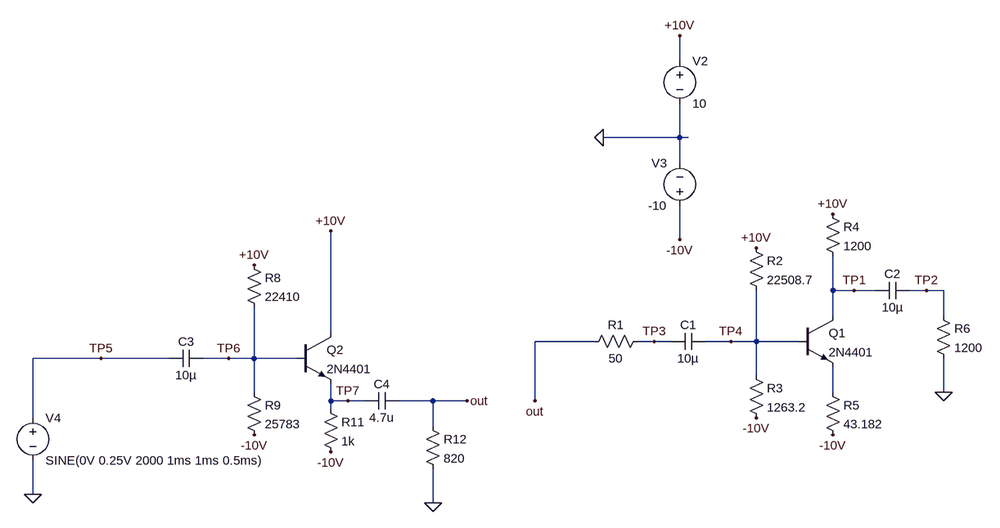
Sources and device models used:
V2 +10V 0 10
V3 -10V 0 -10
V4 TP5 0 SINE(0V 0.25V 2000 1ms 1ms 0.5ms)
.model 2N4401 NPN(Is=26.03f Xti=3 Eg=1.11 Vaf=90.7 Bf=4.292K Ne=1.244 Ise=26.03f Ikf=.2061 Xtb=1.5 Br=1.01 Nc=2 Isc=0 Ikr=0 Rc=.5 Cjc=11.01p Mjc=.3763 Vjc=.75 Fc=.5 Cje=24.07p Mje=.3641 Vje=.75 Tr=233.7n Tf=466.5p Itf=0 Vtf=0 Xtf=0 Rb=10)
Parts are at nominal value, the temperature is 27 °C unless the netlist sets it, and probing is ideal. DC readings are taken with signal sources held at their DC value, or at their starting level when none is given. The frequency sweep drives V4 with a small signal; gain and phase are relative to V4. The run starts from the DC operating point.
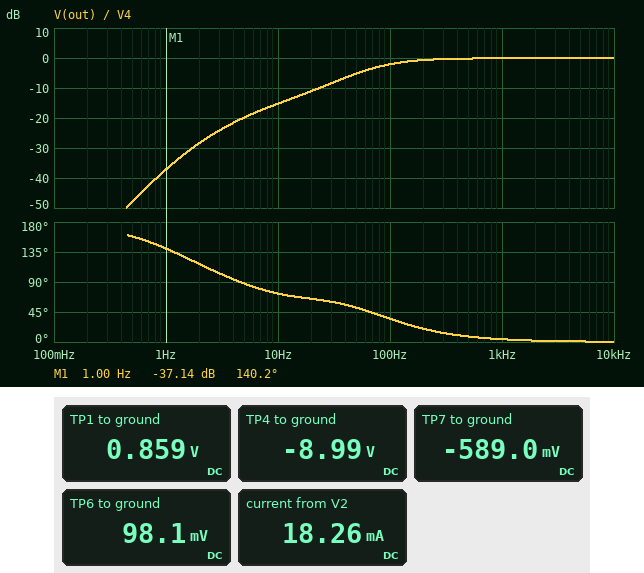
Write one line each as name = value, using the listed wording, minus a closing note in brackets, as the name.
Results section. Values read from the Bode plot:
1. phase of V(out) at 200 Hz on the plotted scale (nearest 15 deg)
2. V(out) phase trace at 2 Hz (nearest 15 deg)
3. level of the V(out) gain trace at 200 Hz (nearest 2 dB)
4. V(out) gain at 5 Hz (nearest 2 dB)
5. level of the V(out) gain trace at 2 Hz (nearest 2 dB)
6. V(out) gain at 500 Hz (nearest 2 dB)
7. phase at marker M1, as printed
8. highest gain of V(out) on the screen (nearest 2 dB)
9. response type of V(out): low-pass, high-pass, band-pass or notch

phase of V(out) at 200 Hz on the plotted scale = 15 deg
V(out) phase trace at 2 Hz = 120 deg
level of the V(out) gain trace at 200 Hz = 0 dB
V(out) gain at 5 Hz = -20 dB
level of the V(out) gain trace at 2 Hz = -28 dB
V(out) gain at 500 Hz = 0 dB
phase at marker M1, as printed = 140.2 deg
highest gain of V(out) on the screen = 0 dB
response type of V(out): low-pass, high-pass, band-pass or notch = high-pass
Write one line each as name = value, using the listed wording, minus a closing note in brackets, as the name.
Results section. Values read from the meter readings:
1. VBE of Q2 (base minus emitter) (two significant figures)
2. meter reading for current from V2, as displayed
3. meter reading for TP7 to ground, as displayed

VBE of Q2 (base minus emitter) = 690 mV
meter reading for current from V2, as displayed = 18.26 mA
meter reading for TP7 to ground, as displayed = -589.0 mV
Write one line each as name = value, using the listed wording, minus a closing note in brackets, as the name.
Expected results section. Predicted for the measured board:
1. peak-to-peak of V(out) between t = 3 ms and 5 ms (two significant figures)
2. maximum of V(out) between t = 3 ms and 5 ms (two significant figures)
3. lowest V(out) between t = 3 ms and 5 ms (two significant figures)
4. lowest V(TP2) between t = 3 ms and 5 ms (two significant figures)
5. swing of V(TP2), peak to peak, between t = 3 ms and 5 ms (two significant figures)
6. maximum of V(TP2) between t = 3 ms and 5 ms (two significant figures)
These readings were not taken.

peak-to-peak of V(out) between t = 3 ms and 5 ms = 500 mV
maximum of V(out) between t = 3 ms and 5 ms = 250 mV
lowest V(out) between t = 3 ms and 5 ms = -250 mV
lowest V(TP2) between t = 3 ms and 5 ms = -3.0 V
swing of V(TP2), peak to peak, between t = 3 ms and 5 ms = 6.0 V
maximum of V(TP2) between t = 3 ms and 5 ms = 2.9 V
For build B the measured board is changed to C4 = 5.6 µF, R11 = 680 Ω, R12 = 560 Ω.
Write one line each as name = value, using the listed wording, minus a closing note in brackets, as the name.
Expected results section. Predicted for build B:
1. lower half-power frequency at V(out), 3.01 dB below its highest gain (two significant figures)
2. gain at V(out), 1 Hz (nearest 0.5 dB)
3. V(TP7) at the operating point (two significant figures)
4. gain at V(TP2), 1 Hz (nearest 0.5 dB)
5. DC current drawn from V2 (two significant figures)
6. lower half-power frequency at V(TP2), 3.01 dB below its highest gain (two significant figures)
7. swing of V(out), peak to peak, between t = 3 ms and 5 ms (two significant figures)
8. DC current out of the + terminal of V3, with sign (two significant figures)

lower half-power frequency at V(out), 3.01 dB below its highest gain = 80 Hz
gain at V(out), 1 Hz = -39.0 dB
V(TP7) at the operating point = -810 mV
gain at V(TP2), 1 Hz = -57.0 dB
DC current drawn from V2 = 22 mA
lower half-power frequency at V(TP2), 3.01 dB below its highest gain = 83 Hz
swing of V(out), peak to peak, between t = 3 ms and 5 ms = 500 mV
DC current out of the + terminal of V3, with sign = -22 mA
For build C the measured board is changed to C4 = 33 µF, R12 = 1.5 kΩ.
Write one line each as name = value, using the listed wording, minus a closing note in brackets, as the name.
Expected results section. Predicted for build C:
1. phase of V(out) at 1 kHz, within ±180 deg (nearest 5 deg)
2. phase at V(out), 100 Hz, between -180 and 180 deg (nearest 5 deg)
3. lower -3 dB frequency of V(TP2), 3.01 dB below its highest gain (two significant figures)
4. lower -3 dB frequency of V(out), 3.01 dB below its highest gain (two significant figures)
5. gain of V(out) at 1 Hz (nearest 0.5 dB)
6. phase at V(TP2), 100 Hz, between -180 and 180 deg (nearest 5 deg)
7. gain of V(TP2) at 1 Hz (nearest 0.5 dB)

phase of V(out) at 1 kHz, within ±180 deg = 0 deg
phase at V(out), 100 Hz, between -180 and 180 deg = 5 deg
lower -3 dB frequency of V(TP2), 3.01 dB below its highest gain = 22 Hz
lower -3 dB frequency of V(out), 3.01 dB below its highest gain = 6.8 Hz
gain of V(out) at 1 Hz = -15.5 dB
phase at V(TP2), 100 Hz, between -180 and 180 deg = -165 deg
gain of V(TP2) at 1 Hz = -33.5 dB
